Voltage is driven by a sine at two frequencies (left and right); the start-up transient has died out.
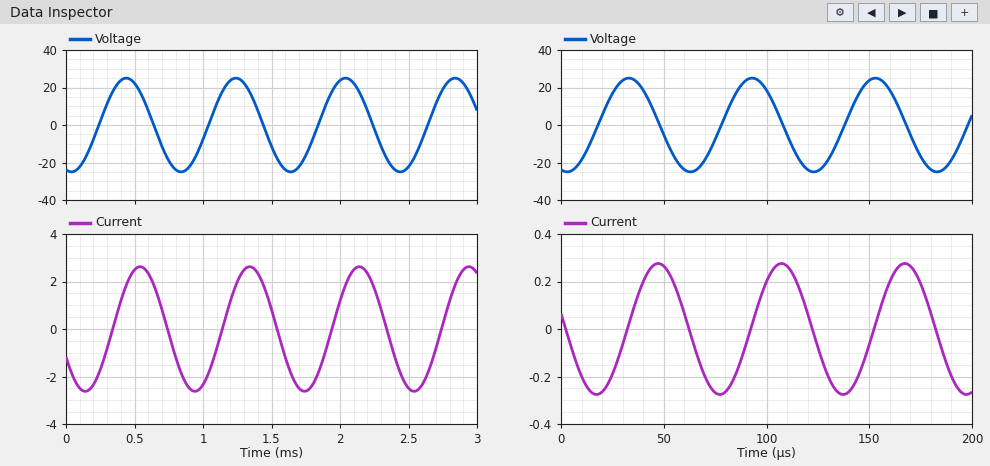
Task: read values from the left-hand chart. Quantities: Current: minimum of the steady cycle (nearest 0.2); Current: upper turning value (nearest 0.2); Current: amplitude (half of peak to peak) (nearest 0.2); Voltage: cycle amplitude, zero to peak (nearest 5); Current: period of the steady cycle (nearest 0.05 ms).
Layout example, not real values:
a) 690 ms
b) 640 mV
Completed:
a) -2.6
b) 2.6
c) 2.6
d) 25
e) 0.80 ms
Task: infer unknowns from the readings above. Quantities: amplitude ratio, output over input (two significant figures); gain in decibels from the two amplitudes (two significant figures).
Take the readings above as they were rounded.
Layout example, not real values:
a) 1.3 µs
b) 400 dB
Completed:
a) 0.10
b) -20 dB
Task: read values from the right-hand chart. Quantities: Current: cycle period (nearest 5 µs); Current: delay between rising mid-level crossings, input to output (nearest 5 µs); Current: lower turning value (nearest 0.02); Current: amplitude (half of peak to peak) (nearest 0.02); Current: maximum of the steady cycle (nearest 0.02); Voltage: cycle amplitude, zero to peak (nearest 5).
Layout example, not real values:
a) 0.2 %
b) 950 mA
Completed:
a) 60 µs
b) 15 µs
c) -0.28
d) 0.28
e) 0.28
f) 25
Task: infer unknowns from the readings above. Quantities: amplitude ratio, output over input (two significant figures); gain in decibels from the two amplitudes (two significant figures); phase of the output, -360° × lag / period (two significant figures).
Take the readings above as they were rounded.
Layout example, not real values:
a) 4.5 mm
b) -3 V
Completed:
a) 0.011
b) -39 dB
c) -90°
